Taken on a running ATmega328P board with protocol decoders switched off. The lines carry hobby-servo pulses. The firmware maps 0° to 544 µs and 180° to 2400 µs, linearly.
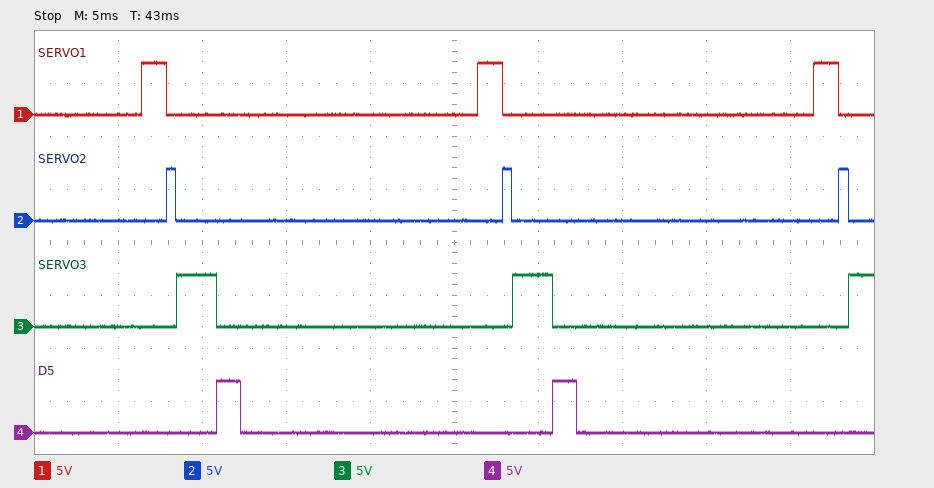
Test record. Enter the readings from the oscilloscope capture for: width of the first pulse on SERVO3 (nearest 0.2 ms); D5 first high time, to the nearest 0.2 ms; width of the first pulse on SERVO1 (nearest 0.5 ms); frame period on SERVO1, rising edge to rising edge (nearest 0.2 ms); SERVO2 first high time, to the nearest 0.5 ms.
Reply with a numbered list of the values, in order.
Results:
1. 2.4 ms
2. 1.4 ms
3. 1.5 ms
4. 20.0 ms
5. 0.5 ms
